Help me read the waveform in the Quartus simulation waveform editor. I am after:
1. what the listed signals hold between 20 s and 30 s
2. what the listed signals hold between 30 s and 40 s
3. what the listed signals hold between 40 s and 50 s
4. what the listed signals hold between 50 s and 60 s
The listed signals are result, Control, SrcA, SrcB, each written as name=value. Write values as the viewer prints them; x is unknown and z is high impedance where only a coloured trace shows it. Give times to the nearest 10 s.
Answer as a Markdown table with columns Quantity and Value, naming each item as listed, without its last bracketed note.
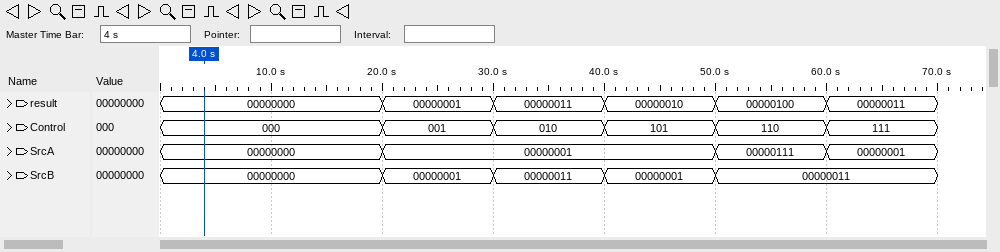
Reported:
| Quantity | Value |
|---|---|
| what the listed signals hold between 20 s and 30 s | result=00000001, Control=001, SrcA=00000001, SrcB=00000001 |
| what the listed signals hold between 30 s and 40 s | result=00000011, Control=010, SrcA=00000001, SrcB=00000011 |
| what the listed signals hold between 40 s and 50 s | result=00000010, Control=101, SrcA=00000001, SrcB=00000001 |
| what the listed signals hold between 50 s and 60 s | result=00000100, Control=110, SrcA=00000111, SrcB=00000011 |
